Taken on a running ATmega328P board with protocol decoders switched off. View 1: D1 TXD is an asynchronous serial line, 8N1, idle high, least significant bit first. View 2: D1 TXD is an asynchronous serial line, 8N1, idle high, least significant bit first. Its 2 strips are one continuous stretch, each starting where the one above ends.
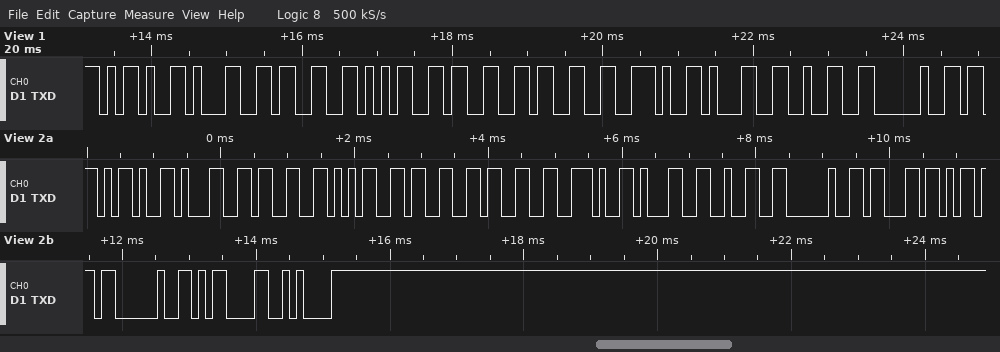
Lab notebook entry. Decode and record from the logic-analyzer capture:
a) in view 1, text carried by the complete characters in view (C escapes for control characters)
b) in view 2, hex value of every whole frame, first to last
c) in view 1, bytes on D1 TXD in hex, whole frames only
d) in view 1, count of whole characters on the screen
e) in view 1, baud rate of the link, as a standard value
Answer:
"-13533.12 "
2D 31 33 35 33 33 2E 31 32 20 63 6D 20 0D 0A
2D 31 33 35 33 33 2E 31 32 20
10
9600 baud
